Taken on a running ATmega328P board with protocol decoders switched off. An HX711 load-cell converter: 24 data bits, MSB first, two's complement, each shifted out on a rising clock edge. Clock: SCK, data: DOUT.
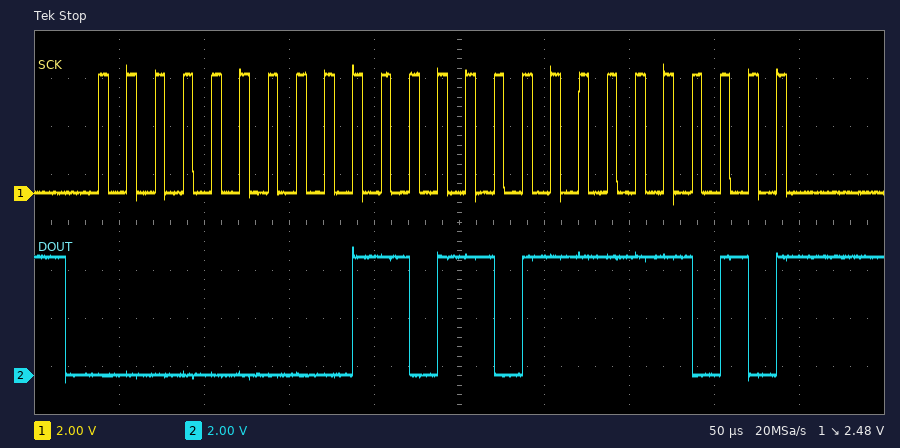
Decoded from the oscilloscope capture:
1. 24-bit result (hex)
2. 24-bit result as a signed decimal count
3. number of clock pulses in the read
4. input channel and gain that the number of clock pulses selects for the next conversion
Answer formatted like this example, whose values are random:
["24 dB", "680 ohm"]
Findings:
["0x006DFA", "28154", "25", "channel A, gain 128"]
